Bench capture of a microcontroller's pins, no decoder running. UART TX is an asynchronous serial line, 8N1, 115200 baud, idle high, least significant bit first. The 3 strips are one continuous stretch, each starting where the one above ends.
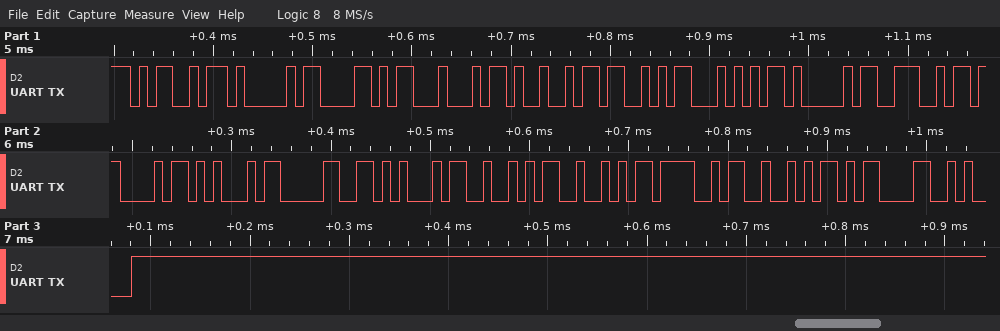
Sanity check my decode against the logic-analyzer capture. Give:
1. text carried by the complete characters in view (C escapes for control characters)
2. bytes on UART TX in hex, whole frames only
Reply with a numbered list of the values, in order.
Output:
1. "MAXDISTANCE0ERROR\r\n"
2. 4D 41 58 44 49 53 54 41 4E 43 45 30 45 52 52 4F 52 0D 0A
